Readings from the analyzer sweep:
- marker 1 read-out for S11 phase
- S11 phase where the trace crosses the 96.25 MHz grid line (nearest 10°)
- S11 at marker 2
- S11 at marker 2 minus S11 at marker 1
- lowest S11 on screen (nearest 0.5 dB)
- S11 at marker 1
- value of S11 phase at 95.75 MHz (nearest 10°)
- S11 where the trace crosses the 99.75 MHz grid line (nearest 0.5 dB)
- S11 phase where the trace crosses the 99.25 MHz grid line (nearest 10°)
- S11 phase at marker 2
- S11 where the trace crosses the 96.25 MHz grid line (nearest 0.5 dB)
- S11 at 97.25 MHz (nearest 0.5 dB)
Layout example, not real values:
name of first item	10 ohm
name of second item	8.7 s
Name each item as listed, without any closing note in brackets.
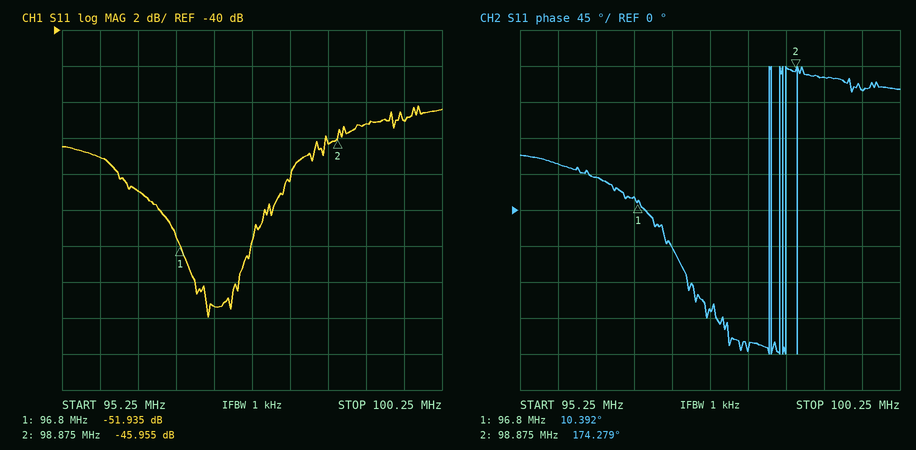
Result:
marker 1 read-out for S11 phase	10.392°
S11 phase where the trace crosses the 96.25 MHz grid line	40°
S11 at marker 2	-45.955 dB
S11 at marker 2 minus S11 at marker 1	5.980 dB
lowest S11 on screen	-56.0 dB
S11 at marker 1	-51.935 dB
value of S11 phase at 95.75 MHz	60°
S11 where the trace crosses the 99.75 MHz grid line	-45.0 dB
S11 phase where the trace crosses the 99.25 MHz grid line	170°
S11 phase at marker 2	174.279°
S11 where the trace crosses the 96.25 MHz grid line	-49.0 dB
S11 at 97.25 MHz	-55.5 dB
